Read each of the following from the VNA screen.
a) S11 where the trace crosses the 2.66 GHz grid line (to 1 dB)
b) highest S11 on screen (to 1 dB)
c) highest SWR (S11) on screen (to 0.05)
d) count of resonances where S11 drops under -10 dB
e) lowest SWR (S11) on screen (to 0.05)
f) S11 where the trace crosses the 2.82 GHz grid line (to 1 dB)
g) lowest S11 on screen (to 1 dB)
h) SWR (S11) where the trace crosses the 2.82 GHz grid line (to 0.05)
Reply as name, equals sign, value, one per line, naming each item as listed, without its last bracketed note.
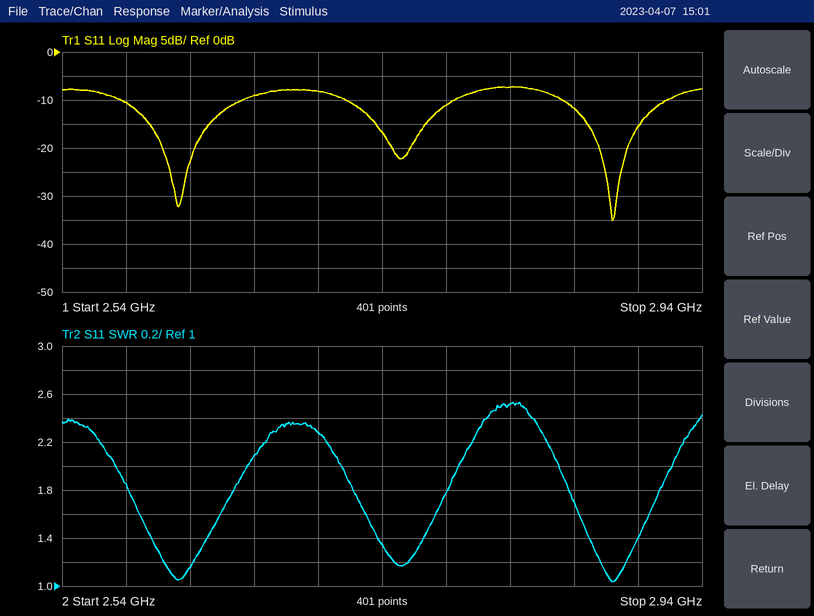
S11 where the trace crosses the 2.66 GHz grid line = -9 dB
highest S11 on screen = -7 dB
highest SWR (S11) on screen = 2.55
count of resonances where S11 drops under -10 dB = 3
lowest SWR (S11) on screen = 1.05
S11 where the trace crosses the 2.82 GHz grid line = -7 dB
lowest S11 on screen = -35 dB
SWR (S11) where the trace crosses the 2.82 GHz grid line = 2.50
